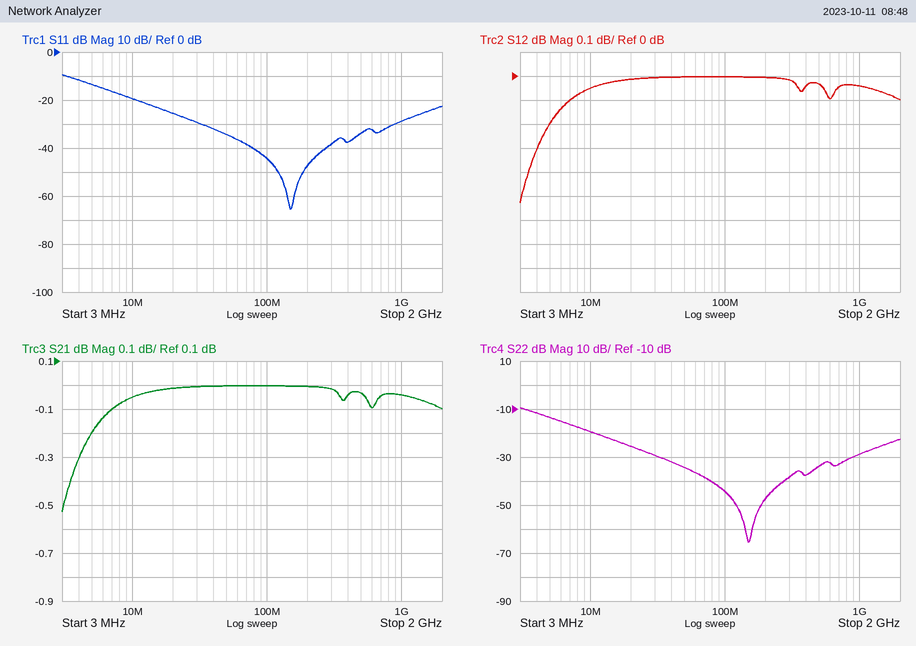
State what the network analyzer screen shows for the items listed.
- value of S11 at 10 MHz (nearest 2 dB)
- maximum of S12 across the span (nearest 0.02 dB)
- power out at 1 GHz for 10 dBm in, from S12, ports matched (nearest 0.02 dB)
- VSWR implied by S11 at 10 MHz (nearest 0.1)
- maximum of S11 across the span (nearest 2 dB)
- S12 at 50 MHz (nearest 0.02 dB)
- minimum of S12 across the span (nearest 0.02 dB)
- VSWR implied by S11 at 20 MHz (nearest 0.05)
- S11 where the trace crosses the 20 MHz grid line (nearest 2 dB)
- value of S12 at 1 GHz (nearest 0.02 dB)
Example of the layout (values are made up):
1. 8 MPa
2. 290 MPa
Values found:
1. -20 dB
2. 0.00 dB
3. 9.96 dBm
4. 1.2
5. -10 dB
6. 0.00 dB
7. -0.52 dB
8. 1.10
9. -26 dB
10. -0.04 dB
